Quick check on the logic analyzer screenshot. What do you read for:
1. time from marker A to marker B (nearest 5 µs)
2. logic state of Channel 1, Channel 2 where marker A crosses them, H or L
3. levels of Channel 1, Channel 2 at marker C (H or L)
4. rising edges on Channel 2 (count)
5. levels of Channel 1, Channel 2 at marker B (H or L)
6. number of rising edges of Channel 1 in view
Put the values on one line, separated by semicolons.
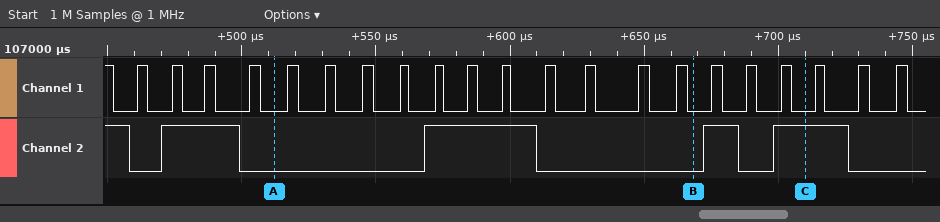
155 µs; Channel 1=L, Channel 2=L; Channel 1=L, Channel 2=H; 4; Channel 1=L, Channel 2=L; 21
